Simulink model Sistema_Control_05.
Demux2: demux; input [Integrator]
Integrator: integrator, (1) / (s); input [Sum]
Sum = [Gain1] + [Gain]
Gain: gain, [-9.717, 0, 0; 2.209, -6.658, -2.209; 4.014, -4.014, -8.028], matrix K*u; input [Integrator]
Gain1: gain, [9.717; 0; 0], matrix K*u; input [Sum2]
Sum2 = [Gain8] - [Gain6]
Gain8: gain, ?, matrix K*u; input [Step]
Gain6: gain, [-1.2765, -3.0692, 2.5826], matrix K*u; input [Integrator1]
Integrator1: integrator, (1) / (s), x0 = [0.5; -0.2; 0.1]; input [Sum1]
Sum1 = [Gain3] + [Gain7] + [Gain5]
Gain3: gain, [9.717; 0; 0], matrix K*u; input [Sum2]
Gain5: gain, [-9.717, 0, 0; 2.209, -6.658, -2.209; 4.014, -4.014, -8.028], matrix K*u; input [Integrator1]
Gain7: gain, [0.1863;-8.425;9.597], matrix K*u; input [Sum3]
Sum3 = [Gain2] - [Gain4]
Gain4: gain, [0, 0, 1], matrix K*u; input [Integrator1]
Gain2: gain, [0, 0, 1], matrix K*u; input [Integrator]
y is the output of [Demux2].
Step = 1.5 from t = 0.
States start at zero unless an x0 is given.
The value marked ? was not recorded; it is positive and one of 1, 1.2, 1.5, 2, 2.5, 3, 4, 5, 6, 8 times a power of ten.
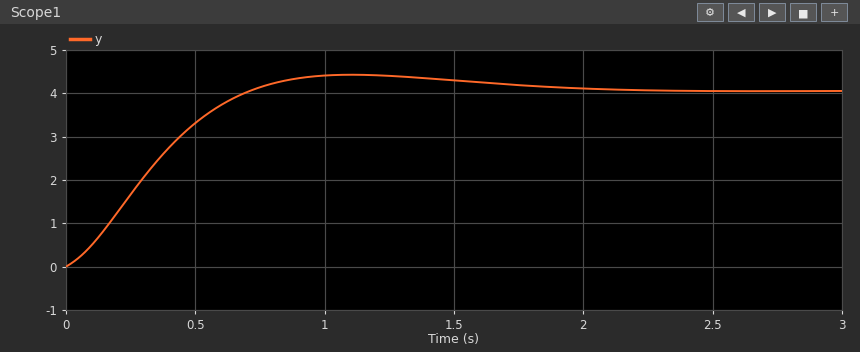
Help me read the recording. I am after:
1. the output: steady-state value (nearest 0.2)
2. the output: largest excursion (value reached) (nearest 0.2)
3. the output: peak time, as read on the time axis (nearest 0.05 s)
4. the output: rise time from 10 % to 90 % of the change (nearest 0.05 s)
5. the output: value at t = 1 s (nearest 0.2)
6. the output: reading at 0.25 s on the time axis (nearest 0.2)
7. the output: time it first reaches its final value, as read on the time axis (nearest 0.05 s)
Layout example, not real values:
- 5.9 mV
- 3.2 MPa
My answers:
- 4.0
- 4.4
- 1.10 s
- 0.50 s
- 4.4
- 1.6
- 0.70 s
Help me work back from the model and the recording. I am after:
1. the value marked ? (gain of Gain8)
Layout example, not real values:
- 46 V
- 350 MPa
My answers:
- 0.4
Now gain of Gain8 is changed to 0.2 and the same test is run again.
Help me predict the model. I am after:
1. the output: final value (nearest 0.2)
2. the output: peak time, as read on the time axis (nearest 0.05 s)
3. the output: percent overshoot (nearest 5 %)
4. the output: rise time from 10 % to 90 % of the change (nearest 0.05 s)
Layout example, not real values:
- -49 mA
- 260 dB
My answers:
- 2.0
- 1.00 s
- 15 %
- 0.40 s
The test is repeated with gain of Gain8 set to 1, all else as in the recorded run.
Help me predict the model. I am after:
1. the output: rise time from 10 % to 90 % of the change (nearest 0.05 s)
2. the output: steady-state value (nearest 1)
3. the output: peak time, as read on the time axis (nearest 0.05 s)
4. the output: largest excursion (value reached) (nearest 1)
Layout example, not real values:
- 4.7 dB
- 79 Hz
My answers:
- 0.55 s
- 10
- 1.20 s
- 11
